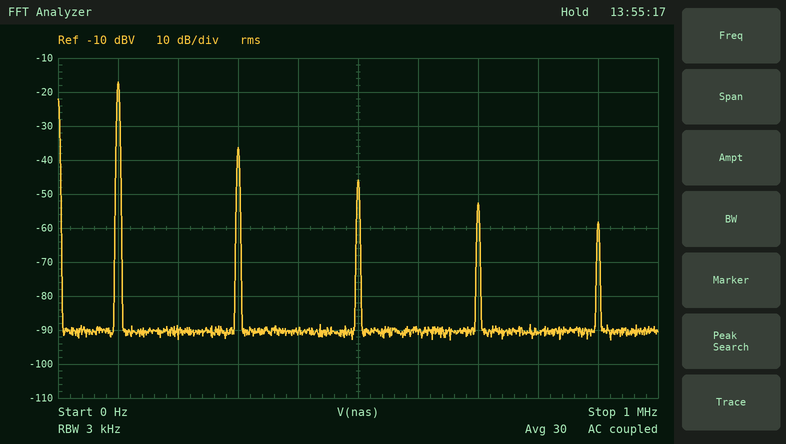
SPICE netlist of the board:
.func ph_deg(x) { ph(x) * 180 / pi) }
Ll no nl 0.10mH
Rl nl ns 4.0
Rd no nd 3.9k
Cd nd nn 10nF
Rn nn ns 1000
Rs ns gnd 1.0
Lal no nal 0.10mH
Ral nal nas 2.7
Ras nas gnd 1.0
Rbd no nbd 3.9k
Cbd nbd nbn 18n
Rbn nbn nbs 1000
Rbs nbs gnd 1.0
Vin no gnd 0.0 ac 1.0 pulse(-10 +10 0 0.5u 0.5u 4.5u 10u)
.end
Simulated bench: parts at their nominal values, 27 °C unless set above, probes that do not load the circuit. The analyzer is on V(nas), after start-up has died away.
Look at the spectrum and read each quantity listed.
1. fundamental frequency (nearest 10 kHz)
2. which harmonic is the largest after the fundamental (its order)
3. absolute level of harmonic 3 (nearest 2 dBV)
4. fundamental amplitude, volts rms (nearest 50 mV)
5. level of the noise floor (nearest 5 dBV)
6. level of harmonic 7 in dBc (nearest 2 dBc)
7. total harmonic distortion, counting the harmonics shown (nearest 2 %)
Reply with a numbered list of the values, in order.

1. 100 kHz
2. 3
3. -36 dBV
4. 150 mV
5. -90 dBV
6. -36 dBc
7. 12 %
